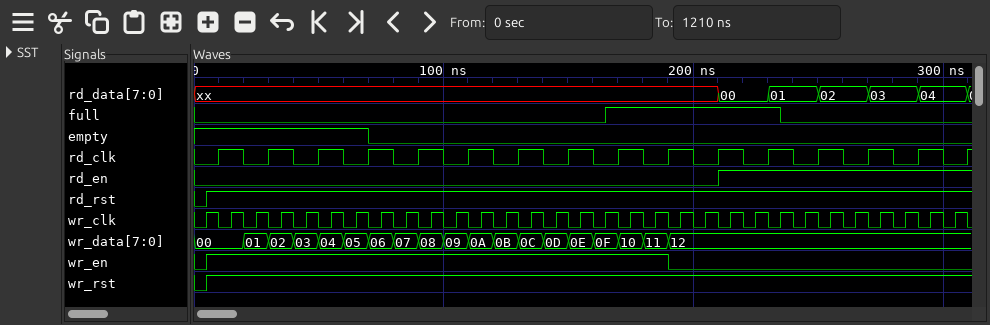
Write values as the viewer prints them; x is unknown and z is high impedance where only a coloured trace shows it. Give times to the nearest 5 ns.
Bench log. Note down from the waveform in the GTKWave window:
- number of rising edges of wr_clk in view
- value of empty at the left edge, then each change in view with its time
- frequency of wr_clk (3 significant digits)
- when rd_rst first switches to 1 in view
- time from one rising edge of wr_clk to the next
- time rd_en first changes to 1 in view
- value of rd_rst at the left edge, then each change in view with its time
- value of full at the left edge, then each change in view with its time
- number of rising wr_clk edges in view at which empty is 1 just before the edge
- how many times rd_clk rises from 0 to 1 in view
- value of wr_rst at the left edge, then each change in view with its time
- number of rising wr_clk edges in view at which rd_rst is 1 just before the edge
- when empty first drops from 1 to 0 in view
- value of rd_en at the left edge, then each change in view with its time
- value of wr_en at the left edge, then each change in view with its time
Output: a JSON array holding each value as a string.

["31", "1, 0 at 70 ns", "100 MHz", "5 ns", "10 ns", "210 ns", "0, 1 at 5 ns", "0, 1 at 165 ns, 0 at 235 ns", "7", "16", "0, 1 at 5 ns", "30", "70 ns", "0, 1 at 210 ns", "0, 1 at 5 ns, 0 at 190 ns"]
